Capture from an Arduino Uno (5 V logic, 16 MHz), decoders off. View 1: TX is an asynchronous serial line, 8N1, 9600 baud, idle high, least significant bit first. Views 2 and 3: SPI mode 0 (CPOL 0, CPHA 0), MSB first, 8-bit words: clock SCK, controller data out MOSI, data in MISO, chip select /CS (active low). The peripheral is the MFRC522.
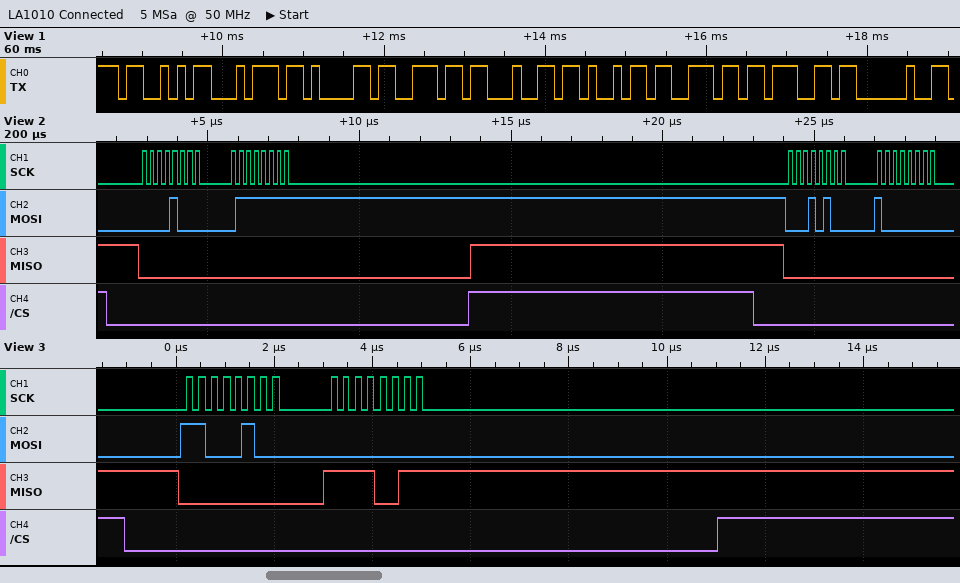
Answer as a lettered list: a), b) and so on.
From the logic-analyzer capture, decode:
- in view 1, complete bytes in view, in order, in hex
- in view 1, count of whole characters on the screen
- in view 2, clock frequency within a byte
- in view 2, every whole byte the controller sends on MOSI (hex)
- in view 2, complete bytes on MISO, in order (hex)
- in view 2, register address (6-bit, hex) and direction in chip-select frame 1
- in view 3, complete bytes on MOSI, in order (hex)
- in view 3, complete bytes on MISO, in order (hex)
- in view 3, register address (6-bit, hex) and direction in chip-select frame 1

a) 53 74 61 6E 64 69 6E 67 20
b) 9
c) 4 MHz
d) 08 7F 14 80
e) 00 00 00 00
f) 0x04 write
g) C4 00
h) 00 F3
i) 0x22 read
